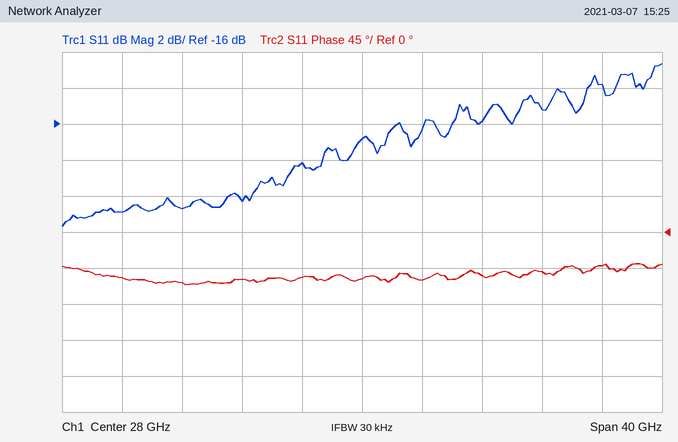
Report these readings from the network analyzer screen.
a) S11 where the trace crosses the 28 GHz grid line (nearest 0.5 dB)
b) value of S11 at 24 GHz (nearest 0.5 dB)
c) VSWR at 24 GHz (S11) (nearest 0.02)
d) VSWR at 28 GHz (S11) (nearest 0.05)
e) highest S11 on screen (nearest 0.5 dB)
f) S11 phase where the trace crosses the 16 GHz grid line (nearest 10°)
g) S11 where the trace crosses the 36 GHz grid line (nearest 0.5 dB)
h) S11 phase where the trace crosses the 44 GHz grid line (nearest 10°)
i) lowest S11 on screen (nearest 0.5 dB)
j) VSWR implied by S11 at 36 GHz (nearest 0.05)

-17.0 dB
-18.0 dB
1.28
1.35
-12.5 dB
-60°
-16.0 dB
-40°
-21.5 dB
1.40
